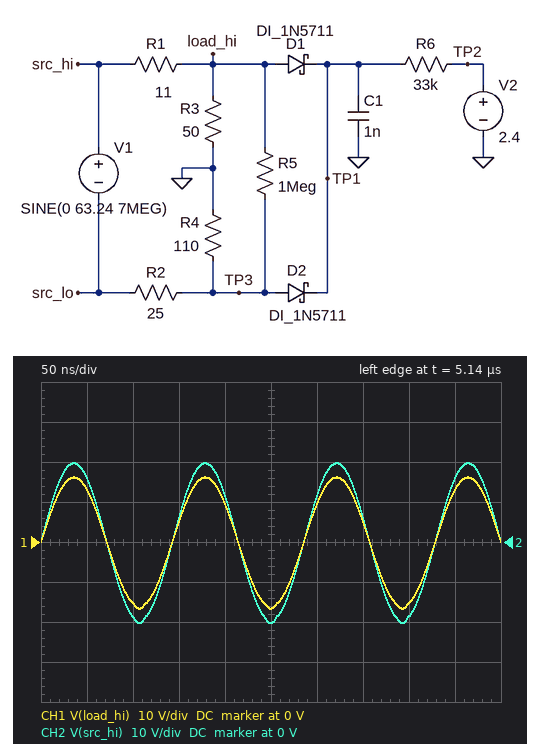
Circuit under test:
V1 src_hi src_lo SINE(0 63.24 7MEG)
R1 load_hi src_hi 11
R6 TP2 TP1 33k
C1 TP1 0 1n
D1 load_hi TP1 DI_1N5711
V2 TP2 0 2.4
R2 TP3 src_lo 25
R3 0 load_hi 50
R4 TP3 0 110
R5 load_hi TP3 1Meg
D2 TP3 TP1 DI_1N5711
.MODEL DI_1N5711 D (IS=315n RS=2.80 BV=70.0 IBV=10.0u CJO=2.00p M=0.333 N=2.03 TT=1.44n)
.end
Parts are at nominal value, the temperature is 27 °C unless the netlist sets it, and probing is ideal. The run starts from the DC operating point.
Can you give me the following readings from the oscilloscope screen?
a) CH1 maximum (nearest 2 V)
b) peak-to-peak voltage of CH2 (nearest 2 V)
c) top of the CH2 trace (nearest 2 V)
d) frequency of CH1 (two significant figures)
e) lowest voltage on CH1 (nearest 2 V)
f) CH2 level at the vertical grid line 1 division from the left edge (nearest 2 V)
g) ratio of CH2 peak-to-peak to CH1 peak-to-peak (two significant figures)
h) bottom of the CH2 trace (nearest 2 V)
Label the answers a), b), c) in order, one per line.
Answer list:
a) 16 V
b) 40 V
c) 20 V
d) 7.0 MHz
e) -16 V
f) 16 V
g) 1.2
h) -20 V
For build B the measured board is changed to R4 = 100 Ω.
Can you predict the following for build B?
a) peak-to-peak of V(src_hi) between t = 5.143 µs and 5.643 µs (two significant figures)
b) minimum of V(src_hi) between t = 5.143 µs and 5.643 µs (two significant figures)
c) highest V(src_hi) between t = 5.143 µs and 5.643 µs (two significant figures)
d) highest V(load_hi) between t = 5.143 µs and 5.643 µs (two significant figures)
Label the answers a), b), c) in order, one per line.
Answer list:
a) 42 V
b) -21 V
c) 21 V
d) 17 V
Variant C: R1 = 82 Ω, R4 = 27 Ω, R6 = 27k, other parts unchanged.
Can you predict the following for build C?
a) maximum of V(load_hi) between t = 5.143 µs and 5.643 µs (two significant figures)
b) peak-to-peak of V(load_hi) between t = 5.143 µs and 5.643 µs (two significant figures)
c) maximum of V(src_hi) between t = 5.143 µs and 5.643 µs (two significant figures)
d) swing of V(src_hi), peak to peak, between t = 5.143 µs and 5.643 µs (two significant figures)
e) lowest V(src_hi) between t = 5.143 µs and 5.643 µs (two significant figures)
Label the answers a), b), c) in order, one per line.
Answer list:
a) 17 V
b) 34 V
c) 45 V
d) 91 V
e) -45 V
